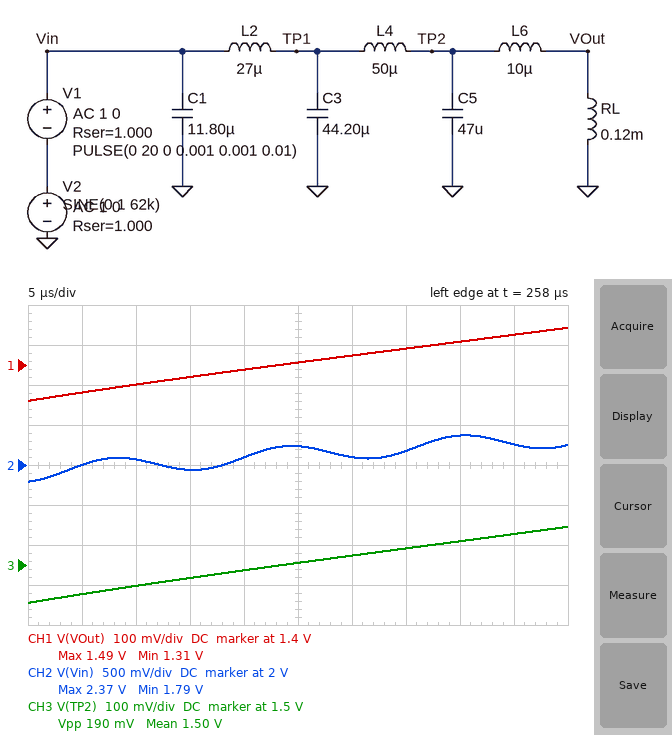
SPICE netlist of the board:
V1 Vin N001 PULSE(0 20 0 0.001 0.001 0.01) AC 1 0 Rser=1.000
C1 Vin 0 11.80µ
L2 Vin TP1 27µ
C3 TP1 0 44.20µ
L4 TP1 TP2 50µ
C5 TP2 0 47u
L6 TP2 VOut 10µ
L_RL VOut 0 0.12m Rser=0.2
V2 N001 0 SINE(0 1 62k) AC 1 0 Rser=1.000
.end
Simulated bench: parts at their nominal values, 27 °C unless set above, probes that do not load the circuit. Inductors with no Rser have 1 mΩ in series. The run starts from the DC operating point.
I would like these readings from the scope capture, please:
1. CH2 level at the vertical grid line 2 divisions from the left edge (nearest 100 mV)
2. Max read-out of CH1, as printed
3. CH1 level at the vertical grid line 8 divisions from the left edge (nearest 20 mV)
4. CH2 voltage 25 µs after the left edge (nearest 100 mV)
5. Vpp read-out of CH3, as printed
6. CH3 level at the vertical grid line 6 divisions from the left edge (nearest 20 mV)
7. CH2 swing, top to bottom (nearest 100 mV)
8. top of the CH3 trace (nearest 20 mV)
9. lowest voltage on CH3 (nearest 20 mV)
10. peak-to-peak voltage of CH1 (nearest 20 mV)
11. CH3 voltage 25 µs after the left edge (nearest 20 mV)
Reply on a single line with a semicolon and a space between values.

2.1 V; 1.49 V; 1.46 V; 2.2 V; 190 mV; 1.52 V; 600 mV; 1.60 V; 1.40 V; 180 mV; 1.50 V
